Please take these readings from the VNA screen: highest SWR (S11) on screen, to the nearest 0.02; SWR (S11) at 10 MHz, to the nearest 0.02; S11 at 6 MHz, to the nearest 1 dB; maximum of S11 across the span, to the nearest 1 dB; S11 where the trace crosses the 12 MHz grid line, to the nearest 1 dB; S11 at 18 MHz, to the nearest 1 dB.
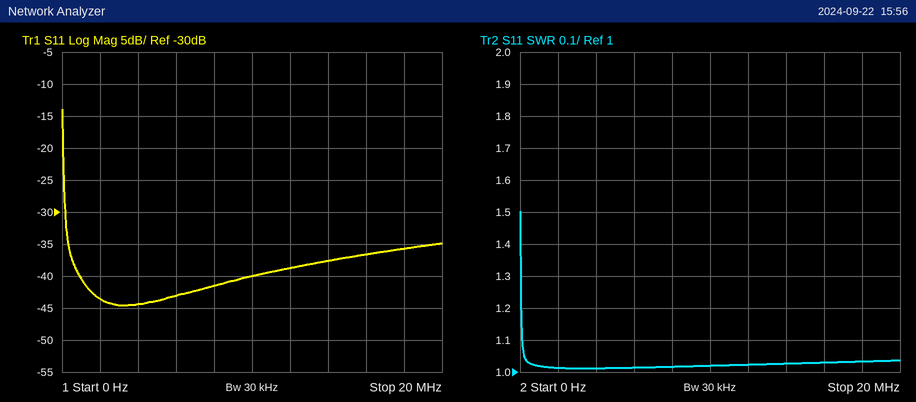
1.50
1.02
-43 dB
-14 dB
-39 dB
-36 dB
